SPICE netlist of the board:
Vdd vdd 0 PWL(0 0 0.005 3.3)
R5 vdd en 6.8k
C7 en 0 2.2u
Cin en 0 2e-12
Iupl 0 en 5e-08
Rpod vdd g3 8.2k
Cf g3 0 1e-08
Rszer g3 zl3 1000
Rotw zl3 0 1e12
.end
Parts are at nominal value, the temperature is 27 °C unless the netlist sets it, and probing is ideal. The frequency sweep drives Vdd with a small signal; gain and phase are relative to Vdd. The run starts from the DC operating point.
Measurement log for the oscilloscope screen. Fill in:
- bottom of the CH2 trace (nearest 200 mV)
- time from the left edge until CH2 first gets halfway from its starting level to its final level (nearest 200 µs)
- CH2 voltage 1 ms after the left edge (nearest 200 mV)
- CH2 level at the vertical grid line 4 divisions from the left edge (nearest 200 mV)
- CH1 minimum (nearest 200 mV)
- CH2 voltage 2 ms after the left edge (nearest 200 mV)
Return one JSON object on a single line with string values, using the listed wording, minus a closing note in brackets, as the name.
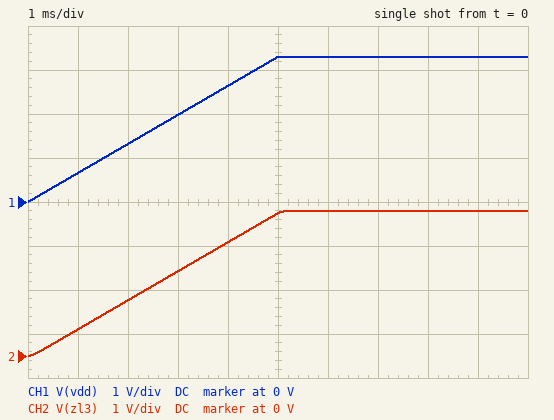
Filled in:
{"bottom of the CH2 trace": "0 V", "time from the left edge until CH2 first gets halfway from its starting level to its final level": "2.6 ms", "CH2 voltage 1 ms after the left edge": "600 mV", "CH2 level at the vertical grid line 4 divisions from the left edge": "2.6 V", "CH1 minimum": "0 V", "CH2 voltage 2 ms after the left edge": "1.2 V"}
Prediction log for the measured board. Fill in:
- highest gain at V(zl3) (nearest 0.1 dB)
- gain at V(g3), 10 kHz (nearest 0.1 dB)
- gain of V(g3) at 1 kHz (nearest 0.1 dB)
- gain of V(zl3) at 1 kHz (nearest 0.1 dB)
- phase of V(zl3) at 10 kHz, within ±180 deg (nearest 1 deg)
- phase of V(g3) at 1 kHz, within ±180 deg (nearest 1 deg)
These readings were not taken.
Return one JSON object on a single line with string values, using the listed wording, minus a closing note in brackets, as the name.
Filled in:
{"highest gain at V(zl3)": "0 dB", "gain at V(g3), 10 kHz": "-14.4 dB", "gain of V(g3) at 1 kHz": "-1.0 dB", "gain of V(zl3) at 1 kHz": "-1.0 dB", "phase of V(zl3) at 10 kHz, within ±180 deg": "-79 deg", "phase of V(g3) at 1 kHz, within ±180 deg": "-27 deg"}
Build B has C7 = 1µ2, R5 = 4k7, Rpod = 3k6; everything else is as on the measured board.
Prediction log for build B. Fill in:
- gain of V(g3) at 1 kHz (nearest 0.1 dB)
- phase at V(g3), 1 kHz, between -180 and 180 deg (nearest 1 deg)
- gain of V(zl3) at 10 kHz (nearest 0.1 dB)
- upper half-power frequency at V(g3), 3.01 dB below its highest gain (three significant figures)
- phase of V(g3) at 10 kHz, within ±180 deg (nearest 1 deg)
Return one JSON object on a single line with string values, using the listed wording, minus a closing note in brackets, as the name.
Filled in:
{"gain of V(g3) at 1 kHz": "-0.2 dB", "phase at V(g3), 1 kHz, between -180 and 180 deg": "-13 deg", "gain of V(zl3) at 10 kHz": "-7.9 dB", "upper half-power frequency at V(g3), 3.01 dB below its highest gain": "4.42 kHz", "phase of V(g3) at 10 kHz, within ±180 deg": "-66 deg"}
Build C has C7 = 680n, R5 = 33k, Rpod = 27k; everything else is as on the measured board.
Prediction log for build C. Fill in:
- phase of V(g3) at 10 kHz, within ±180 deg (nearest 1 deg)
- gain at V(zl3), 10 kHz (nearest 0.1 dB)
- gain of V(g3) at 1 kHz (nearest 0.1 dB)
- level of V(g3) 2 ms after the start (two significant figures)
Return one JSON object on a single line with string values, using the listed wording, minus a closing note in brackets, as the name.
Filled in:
{"phase of V(g3) at 10 kHz, within ±180 deg": "-87 deg", "gain at V(zl3), 10 kHz": "-24.6 dB", "gain of V(g3) at 1 kHz": "-5.9 dB", "level of V(g3) 2 ms after the start": "1.1 V"}
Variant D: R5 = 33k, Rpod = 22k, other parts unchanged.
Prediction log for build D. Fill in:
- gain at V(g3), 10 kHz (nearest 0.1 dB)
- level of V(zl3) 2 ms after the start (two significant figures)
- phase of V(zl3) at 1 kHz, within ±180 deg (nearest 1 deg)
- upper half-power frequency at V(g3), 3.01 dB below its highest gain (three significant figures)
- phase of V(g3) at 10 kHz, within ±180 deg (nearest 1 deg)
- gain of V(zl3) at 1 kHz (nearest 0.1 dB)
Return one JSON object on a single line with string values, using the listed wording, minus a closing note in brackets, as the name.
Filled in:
{"gain at V(g3), 10 kHz": "-22.8 dB", "level of V(zl3) 2 ms after the start": "1.2 V", "phase of V(zl3) at 1 kHz, within ±180 deg": "-54 deg", "upper half-power frequency at V(g3), 3.01 dB below its highest gain": "723 Hz", "phase of V(g3) at 10 kHz, within ±180 deg": "-86 deg", "gain of V(zl3) at 1 kHz": "-4.6 dB"}
